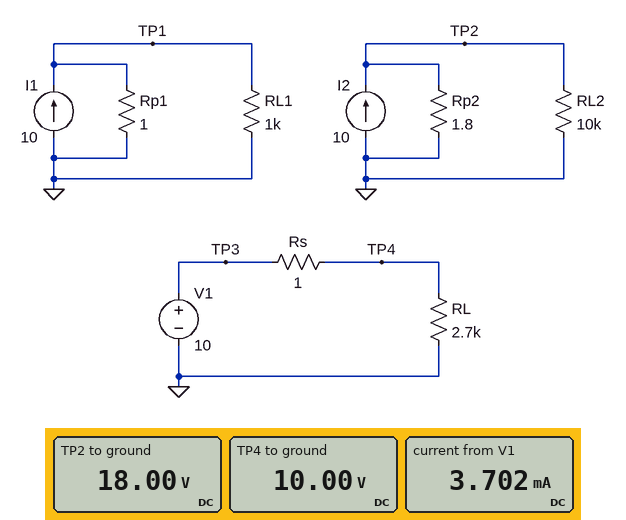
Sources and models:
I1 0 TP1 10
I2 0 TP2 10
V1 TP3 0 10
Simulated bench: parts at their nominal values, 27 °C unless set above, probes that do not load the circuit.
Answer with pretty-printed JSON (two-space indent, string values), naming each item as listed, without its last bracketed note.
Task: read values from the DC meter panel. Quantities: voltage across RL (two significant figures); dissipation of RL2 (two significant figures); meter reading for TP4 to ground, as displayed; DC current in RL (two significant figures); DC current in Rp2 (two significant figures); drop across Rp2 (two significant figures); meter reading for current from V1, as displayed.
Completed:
{
  "voltage across RL": "10 V",
  "dissipation of RL2": "32 mW",
  "meter reading for TP4 to ground, as displayed": "10.00 V",
  "DC current in RL": "3.7 mA",
  "DC current in Rp2": "10 A",
  "drop across Rp2": "18 V",
  "meter reading for current from V1, as displayed": "3.702 mA"
}
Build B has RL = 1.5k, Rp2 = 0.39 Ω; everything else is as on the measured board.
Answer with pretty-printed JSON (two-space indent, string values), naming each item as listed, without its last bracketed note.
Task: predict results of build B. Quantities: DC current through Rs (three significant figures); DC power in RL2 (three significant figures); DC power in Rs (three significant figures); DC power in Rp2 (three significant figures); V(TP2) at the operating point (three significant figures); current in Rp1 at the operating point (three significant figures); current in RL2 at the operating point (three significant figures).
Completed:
{
  "DC current through Rs": "6.66 mA",
  "DC power in RL2": "1.52 mW",
  "DC power in Rs": "44.4 µW",
  "DC power in Rp2": "39.0 W",
  "V(TP2) at the operating point": "3.90 V",
  "current in Rp1 at the operating point": "9.99 A",
  "current in RL2 at the operating point": "390 µA"
}
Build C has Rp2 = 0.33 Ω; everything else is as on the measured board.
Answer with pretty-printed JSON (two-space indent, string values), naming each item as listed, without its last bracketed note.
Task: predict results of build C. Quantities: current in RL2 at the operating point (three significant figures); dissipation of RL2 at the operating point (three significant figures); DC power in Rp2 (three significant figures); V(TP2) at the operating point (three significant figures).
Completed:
{
  "current in RL2 at the operating point": "330 µA",
  "dissipation of RL2 at the operating point": "1.09 mW",
  "DC power in Rp2": "33.0 W",
  "V(TP2) at the operating point": "3.30 V"
}
